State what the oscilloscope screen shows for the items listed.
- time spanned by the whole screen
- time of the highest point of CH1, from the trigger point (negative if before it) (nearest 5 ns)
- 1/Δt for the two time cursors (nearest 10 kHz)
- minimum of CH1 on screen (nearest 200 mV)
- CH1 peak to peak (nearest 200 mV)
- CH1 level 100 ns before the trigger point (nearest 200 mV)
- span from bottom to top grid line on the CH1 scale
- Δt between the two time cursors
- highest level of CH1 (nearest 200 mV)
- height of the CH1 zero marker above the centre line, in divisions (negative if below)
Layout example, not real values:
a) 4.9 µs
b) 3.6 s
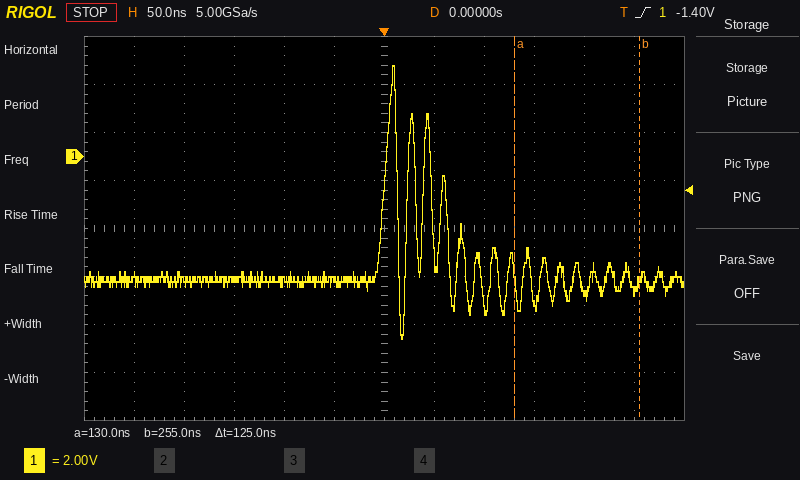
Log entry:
a) 600 ns
b) +10 ns
c) 8.00 MHz
d) -7.6 V
e) 11.4 V
f) -5.2 V
g) 16 V
h) 125 ns
i) 3.8 V
j) +1.5 div
